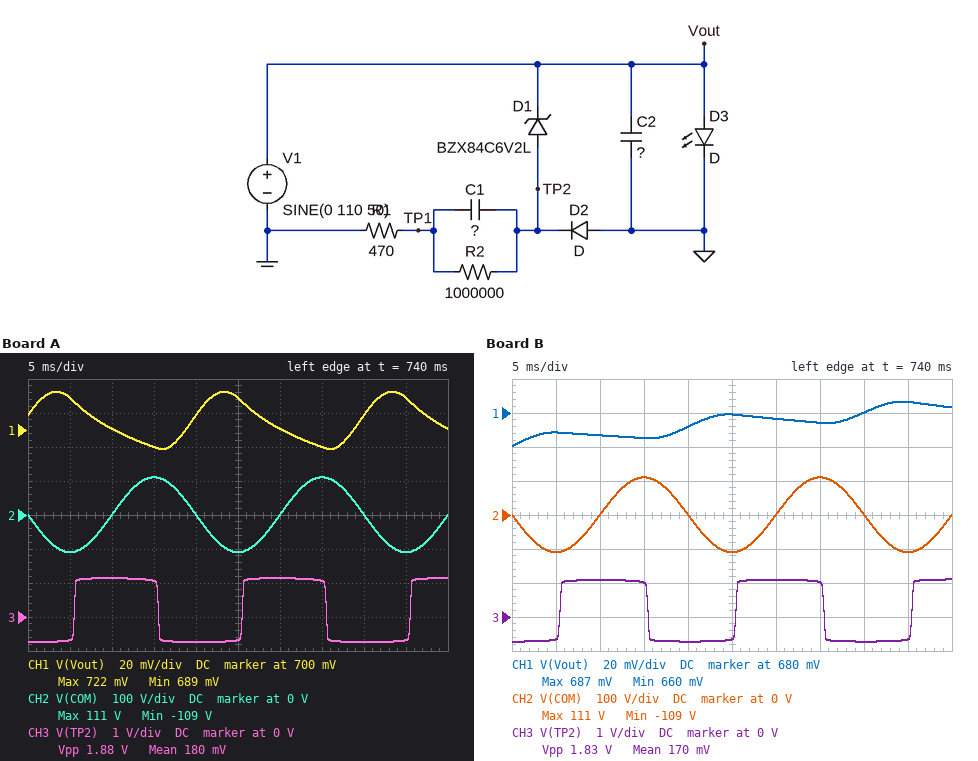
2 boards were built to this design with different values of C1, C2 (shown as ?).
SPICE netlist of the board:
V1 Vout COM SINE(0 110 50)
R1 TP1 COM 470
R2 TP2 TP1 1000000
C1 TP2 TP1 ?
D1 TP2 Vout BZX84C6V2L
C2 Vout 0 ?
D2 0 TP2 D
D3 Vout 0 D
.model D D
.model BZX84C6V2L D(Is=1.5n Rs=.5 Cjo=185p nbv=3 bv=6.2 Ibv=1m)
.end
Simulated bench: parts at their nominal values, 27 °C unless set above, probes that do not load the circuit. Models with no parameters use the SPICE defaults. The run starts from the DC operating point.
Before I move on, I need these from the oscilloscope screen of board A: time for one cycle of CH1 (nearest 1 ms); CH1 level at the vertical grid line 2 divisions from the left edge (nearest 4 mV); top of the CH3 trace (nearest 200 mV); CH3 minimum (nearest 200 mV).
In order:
20 ms
700 mV
1.2 V
-800 mV
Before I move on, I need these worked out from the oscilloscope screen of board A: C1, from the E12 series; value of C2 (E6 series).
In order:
680 nF
2.2 mF
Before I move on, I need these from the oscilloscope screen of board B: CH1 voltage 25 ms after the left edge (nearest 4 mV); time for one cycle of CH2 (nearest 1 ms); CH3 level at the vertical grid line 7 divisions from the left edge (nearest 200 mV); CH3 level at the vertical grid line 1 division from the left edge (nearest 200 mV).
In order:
680 mV
20 ms
1.0 V
-600 mV
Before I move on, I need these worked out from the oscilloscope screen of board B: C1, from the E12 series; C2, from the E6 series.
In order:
390 nF
4.7 mF
